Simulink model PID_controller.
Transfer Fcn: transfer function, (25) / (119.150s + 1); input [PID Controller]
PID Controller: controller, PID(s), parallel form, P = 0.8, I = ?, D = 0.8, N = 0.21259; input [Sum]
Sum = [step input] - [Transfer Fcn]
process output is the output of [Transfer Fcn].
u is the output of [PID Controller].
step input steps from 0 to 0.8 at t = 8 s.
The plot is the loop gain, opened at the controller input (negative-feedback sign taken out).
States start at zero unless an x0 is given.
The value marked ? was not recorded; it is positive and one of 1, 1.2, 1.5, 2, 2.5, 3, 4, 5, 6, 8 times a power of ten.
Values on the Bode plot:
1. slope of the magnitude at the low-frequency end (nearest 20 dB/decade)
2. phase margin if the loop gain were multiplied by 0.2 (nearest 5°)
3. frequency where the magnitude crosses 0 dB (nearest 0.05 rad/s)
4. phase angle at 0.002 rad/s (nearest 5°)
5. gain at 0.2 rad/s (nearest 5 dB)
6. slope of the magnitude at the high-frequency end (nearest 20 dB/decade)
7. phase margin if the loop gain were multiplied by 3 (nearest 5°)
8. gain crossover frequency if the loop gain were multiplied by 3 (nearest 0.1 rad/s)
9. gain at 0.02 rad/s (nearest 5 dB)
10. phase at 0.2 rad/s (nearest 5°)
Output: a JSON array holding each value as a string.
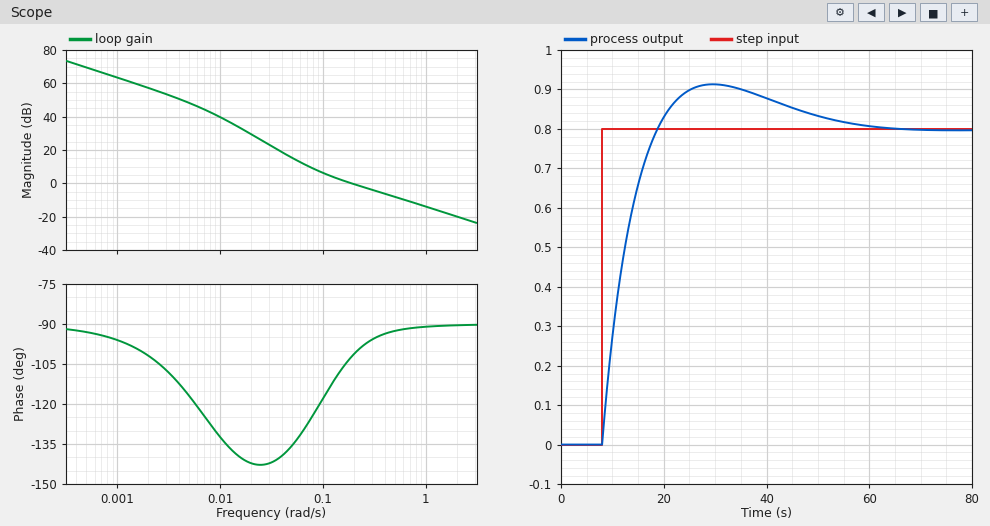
["-20 dB/decade", "45°", "0.20 rad/s", "-100°", "0 dB", "-20 dB/decade", "90°", "0.6 rad/s", "30 dB", "-100°"]
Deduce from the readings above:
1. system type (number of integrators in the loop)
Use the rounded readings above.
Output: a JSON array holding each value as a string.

["1"]
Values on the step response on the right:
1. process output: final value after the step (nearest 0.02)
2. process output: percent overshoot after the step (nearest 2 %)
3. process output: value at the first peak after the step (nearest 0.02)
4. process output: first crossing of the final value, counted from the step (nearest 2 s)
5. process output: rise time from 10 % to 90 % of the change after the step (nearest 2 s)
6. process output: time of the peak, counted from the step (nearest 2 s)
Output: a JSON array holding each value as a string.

["0.80", "14 %", "0.92", "10 s", "8 s", "22 s"]
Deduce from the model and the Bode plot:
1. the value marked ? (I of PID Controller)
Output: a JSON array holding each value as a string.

["0.06"]
